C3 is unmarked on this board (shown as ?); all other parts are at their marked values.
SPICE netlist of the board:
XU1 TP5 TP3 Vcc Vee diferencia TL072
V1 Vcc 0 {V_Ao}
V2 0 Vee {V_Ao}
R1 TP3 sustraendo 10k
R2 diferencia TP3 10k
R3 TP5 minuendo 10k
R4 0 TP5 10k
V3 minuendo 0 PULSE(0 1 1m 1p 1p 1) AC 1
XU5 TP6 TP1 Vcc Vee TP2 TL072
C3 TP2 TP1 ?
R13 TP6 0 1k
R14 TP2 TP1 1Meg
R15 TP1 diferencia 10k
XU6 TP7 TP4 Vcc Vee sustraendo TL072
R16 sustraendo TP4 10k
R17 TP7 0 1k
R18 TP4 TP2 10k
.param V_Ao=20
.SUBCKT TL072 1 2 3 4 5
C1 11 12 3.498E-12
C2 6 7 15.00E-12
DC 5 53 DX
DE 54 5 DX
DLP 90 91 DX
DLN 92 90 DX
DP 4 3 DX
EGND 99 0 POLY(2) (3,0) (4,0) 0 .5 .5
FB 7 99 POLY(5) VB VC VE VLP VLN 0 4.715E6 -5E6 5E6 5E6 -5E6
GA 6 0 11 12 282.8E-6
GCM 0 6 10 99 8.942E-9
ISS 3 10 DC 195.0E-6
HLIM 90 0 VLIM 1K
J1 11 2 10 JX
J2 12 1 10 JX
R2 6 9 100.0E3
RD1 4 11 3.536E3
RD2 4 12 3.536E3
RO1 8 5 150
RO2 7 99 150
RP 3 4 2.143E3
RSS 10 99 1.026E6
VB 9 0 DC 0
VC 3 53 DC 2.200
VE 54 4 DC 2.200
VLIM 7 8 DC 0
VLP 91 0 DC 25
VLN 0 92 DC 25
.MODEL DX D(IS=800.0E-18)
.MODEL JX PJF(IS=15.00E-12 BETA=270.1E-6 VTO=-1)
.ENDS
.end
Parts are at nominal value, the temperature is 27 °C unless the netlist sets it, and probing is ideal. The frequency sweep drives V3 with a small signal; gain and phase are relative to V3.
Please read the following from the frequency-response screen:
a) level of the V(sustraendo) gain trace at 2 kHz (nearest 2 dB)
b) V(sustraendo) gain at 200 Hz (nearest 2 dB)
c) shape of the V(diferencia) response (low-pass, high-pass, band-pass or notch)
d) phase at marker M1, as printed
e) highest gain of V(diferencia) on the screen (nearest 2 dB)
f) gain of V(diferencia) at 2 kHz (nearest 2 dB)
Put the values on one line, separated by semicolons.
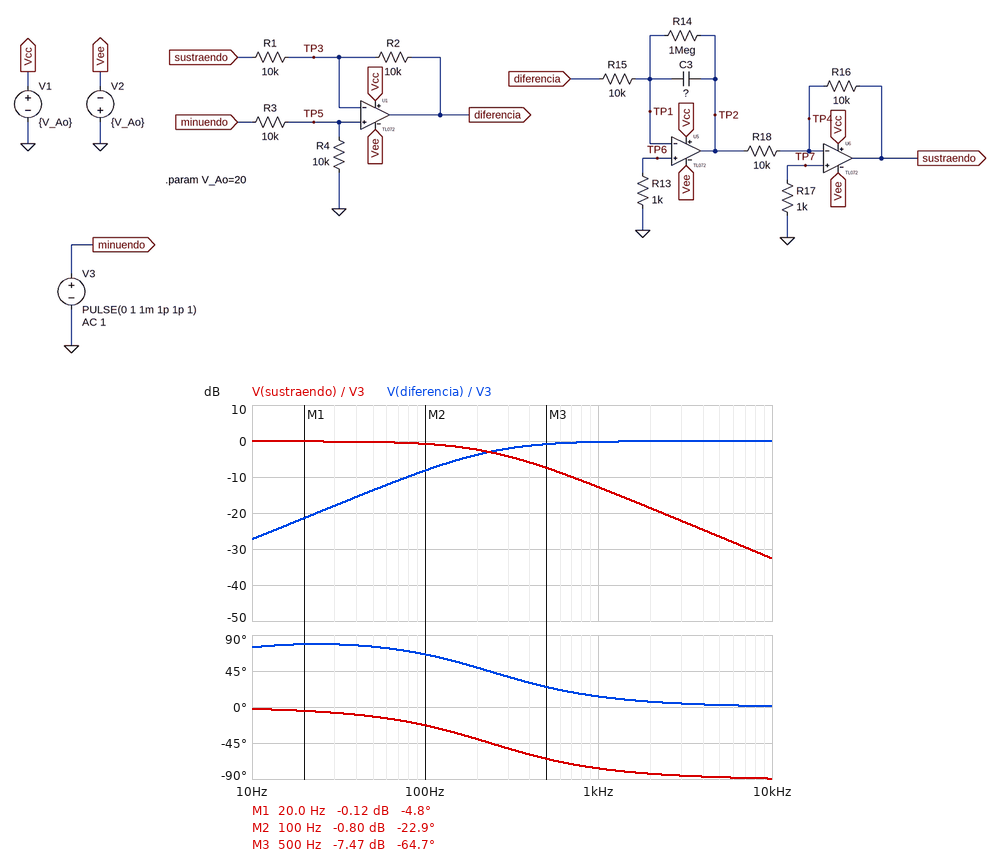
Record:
-18 dB; -2 dB; high-pass; -4.8 deg; 0 dB; 0 dB
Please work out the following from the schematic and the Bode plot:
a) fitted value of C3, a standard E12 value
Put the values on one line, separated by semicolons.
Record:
68 nF
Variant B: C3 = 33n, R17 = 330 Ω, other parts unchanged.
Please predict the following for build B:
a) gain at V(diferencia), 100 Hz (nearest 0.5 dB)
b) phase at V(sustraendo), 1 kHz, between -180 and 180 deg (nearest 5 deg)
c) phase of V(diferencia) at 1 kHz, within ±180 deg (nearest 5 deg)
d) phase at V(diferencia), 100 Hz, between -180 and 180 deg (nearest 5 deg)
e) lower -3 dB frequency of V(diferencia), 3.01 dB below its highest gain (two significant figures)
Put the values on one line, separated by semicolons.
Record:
-14.0 dB; -65 deg; 25 deg; 75 deg; 490 Hz
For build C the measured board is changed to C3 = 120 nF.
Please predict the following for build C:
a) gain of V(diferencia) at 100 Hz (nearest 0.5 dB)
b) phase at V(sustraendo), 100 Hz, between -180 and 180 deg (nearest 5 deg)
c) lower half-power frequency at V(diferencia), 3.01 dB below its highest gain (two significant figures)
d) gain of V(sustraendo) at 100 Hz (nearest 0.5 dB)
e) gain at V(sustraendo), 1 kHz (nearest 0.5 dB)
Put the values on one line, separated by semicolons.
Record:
-4.5 dB; -35 deg; 130 Hz; -2.0 dB; -17.5 dB
